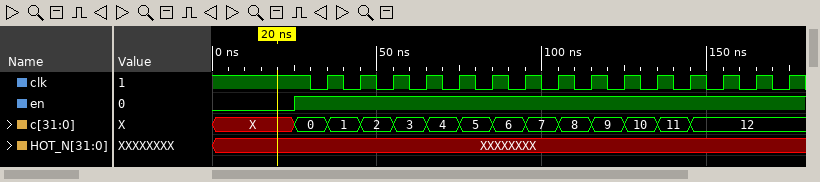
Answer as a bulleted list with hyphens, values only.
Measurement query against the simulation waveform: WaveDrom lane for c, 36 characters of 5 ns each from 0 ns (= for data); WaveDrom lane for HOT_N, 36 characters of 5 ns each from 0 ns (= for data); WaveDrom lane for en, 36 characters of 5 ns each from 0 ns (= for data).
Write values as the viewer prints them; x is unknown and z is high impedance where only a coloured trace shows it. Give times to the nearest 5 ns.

- {name: 'c', wave: 'x....=.=.=.=.=.=.=.=.=.=.=.=.=......', data: '0 1 2 3 4 5 6 7 8 9 10 11 12'}
- {name: 'HOT_N', wave: 'x...................................'}
- {name: 'en', wave: '0....1..............................'}
